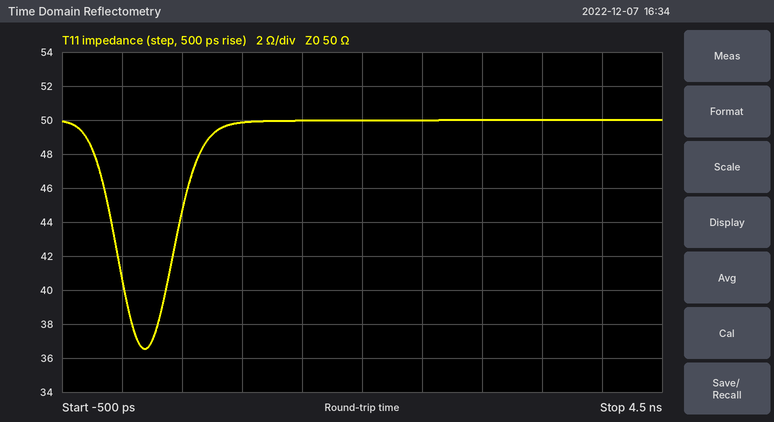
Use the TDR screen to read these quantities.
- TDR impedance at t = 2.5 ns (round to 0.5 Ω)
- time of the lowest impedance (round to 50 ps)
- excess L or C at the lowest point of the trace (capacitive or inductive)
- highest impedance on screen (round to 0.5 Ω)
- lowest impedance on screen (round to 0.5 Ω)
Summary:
50.0 Ω
200 ps
capacitive
50.0 Ω
36.5 Ω
